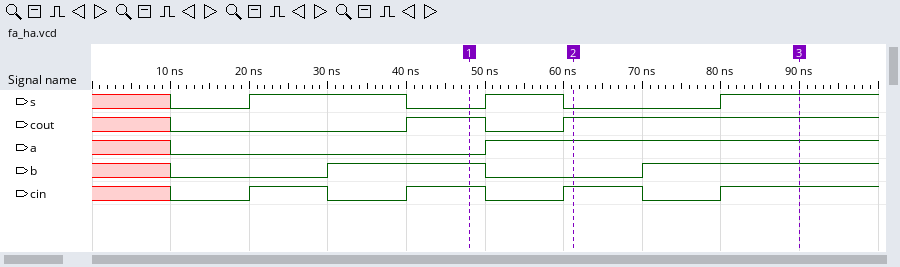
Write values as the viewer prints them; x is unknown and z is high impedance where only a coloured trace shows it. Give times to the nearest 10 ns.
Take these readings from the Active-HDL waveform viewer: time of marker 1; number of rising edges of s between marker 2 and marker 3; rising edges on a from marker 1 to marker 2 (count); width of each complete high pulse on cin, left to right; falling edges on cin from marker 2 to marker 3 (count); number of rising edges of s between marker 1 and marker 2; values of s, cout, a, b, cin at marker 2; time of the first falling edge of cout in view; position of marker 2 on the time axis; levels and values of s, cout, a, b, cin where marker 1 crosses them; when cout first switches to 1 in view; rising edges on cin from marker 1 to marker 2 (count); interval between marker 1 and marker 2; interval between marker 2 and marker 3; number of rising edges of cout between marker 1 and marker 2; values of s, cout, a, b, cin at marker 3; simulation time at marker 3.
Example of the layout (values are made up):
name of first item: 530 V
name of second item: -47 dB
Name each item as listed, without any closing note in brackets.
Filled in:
time of marker 1: 50 ns
number of rising edges of s between marker 2 and marker 3: 1
rising edges on a from marker 1 to marker 2: 1
width of each complete high pulse on cin, left to right: 10 ns, 10 ns, 10 ns
falling edges on cin from marker 2 to marker 3: 1
number of rising edges of s between marker 1 and marker 2: 1
values of s, cout, a, b, cin at marker 2: s=0, cout=1, a=1, b=0, cin=1
time of the first falling edge of cout in view: 50 ns
position of marker 2 on the time axis: 60 ns
levels and values of s, cout, a, b, cin where marker 1 crosses them: s=0, cout=1, a=0, b=1, cin=1
when cout first switches to 1 in view: 40 ns
rising edges on cin from marker 1 to marker 2: 1
interval between marker 1 and marker 2: 10 ns
interval between marker 2 and marker 3: 30 ns
number of rising edges of cout between marker 1 and marker 2: 1
values of s, cout, a, b, cin at marker 3: s=1, cout=1, a=1, b=1, cin=1
simulation time at marker 3: 90 ns
